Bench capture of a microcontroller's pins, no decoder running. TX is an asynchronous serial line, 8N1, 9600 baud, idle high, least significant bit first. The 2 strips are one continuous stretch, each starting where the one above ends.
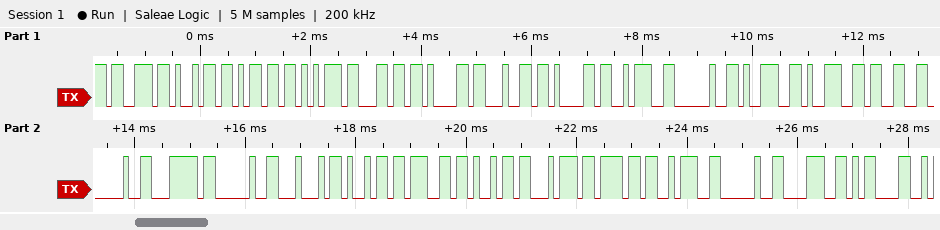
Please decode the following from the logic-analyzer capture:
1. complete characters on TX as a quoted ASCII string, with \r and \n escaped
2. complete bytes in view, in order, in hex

"simulada: 993 | Digito: 8\r"
73 69 6D 75 6C 61 64 61 3A 20 39 39 33 20 7C 20 44 69 67 69 74 6F 3A 20 38 0D
